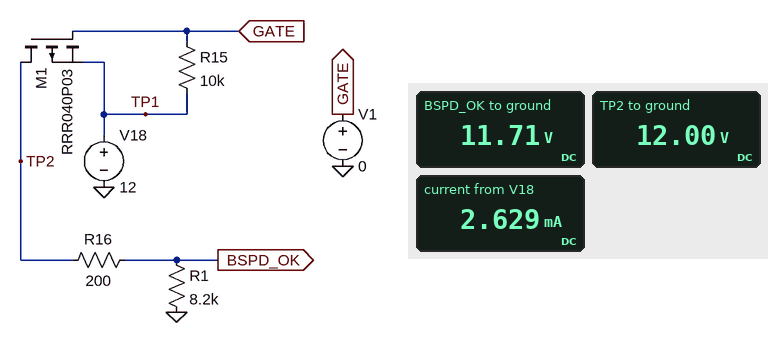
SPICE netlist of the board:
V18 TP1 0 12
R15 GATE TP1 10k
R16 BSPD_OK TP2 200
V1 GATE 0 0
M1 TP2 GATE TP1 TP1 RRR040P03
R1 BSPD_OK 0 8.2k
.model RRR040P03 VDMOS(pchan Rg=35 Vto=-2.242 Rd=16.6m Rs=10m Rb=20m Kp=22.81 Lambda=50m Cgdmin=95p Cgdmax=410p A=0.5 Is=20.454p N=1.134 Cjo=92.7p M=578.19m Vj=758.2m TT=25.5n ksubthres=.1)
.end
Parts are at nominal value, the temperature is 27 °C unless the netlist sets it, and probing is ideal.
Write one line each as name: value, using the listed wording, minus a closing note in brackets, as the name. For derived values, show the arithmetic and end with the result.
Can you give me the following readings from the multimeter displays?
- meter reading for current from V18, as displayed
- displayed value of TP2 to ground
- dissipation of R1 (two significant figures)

meter reading for current from V18, as displayed: 2.629 mA
displayed value of TP2 to ground: 12.00 V
dissipation of R1: (11.71 V)^2 / 8.2 kΩ = 17 mW
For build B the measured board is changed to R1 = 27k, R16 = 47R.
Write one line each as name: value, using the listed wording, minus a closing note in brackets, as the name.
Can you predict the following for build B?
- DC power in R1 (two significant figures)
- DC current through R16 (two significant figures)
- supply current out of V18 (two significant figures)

DC power in R1: 5.3 mW
DC current through R16: 440 µA
supply current out of V18: 1.6 mA
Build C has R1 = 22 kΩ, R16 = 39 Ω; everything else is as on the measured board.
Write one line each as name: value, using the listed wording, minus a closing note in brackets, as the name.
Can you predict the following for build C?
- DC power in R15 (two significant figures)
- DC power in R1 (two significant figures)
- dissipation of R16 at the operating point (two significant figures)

DC power in R15: 14 mW
DC power in R1: 6.5 mW
dissipation of R16 at the operating point: 12 µW
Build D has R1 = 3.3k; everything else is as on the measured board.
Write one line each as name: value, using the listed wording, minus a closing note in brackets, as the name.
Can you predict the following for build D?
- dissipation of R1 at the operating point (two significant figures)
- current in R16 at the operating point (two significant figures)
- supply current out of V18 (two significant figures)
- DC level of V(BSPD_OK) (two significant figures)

dissipation of R1 at the operating point: 39 mW
current in R16 at the operating point: 3.4 mA
supply current out of V18: 4.6 mA
DC level of V(BSPD_OK): 11 V
